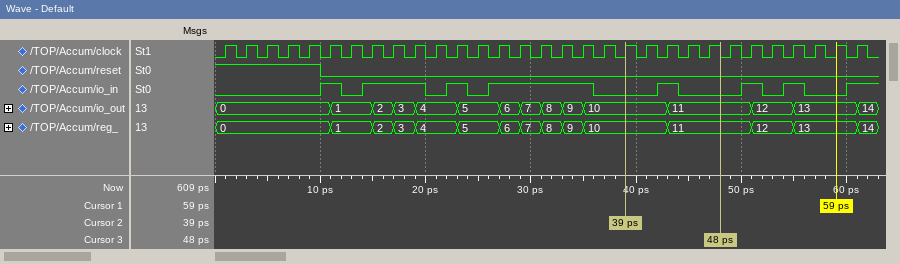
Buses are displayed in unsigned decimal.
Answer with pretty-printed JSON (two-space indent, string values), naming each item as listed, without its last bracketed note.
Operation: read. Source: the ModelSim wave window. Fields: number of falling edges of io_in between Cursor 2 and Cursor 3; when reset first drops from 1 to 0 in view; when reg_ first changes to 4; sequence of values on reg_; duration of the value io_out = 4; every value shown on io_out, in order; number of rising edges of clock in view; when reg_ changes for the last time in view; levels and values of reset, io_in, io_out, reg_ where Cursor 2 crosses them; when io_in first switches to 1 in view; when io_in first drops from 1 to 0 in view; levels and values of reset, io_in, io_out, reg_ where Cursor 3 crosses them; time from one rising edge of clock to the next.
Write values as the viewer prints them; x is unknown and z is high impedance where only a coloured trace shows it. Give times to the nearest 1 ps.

{
  "number of falling edges of io_in between Cursor 2 and Cursor 3": "1",
  "when reset first drops from 1 to 0 in view": "10 ps",
  "when reg_ first changes to 4": "19 ps",
  "sequence of values on reg_": "0, 1, 2, 3, 4, 5, 6, 7, 8, 9, 10, 11, 12, 13, 14",
  "duration of the value io_out = 4": "4 ps",
  "every value shown on io_out, in order": "0, 1, 2, 3, 4, 5, 6, 7, 8, 9, 10, 11, 12, 13, 14",
  "number of rising edges of clock in view": "31",
  "when reg_ changes for the last time in view": "61 ps",
  "levels and values of reset, io_in, io_out, reg_ where Cursor 2 crosses them": "reset=0, io_in=0, io_out=10, reg_=10",
  "when io_in first switches to 1 in view": "10 ps",
  "when io_in first drops from 1 to 0 in view": "12 ps",
  "levels and values of reset, io_in, io_out, reg_ where Cursor 3 crosses them": "reset=0, io_in=0, io_out=11, reg_=11",
  "time from one rising edge of clock to the next": "2 ps"
}
